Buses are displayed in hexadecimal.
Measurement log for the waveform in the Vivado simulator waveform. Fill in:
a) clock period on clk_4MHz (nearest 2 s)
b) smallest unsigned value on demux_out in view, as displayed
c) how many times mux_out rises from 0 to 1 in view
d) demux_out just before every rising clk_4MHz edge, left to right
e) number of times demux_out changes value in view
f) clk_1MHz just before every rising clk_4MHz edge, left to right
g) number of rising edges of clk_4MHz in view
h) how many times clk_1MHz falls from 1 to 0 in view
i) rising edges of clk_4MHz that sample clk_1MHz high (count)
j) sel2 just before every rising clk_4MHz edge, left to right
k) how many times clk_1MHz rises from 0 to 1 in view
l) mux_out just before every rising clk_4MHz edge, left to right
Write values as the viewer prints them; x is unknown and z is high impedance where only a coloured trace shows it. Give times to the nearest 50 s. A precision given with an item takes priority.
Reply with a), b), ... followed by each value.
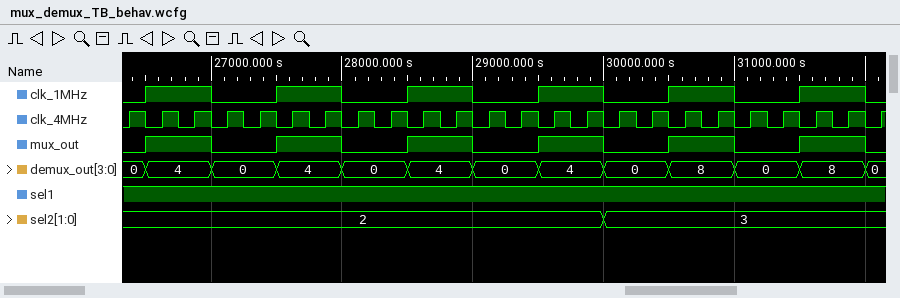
a) 250 s
b) 0
c) 6
d) 0, 4, 4, 0, 0, 4, 4, 0, 0, 4, 4, 0, 0, 4, 4, 0, 0, 8, 8, 0, 0, 8, 8, 0
e) 12
f) 0 1 1 0 0 1 1 0 0 1 1 0 0 1 1 0 0 1 1 0 0 1 1 0
g) 24
h) 6
i) 12
j) 2, 2, 2, 2, 2, 2, 2, 2, 2, 2, 2, 2, 2, 2, 2, 3, 3, 3, 3, 3, 3, 3, 3, 3
k) 6
l) 0 1 1 0 0 1 1 0 0 1 1 0 0 1 1 0 0 1 1 0 0 1 1 0
